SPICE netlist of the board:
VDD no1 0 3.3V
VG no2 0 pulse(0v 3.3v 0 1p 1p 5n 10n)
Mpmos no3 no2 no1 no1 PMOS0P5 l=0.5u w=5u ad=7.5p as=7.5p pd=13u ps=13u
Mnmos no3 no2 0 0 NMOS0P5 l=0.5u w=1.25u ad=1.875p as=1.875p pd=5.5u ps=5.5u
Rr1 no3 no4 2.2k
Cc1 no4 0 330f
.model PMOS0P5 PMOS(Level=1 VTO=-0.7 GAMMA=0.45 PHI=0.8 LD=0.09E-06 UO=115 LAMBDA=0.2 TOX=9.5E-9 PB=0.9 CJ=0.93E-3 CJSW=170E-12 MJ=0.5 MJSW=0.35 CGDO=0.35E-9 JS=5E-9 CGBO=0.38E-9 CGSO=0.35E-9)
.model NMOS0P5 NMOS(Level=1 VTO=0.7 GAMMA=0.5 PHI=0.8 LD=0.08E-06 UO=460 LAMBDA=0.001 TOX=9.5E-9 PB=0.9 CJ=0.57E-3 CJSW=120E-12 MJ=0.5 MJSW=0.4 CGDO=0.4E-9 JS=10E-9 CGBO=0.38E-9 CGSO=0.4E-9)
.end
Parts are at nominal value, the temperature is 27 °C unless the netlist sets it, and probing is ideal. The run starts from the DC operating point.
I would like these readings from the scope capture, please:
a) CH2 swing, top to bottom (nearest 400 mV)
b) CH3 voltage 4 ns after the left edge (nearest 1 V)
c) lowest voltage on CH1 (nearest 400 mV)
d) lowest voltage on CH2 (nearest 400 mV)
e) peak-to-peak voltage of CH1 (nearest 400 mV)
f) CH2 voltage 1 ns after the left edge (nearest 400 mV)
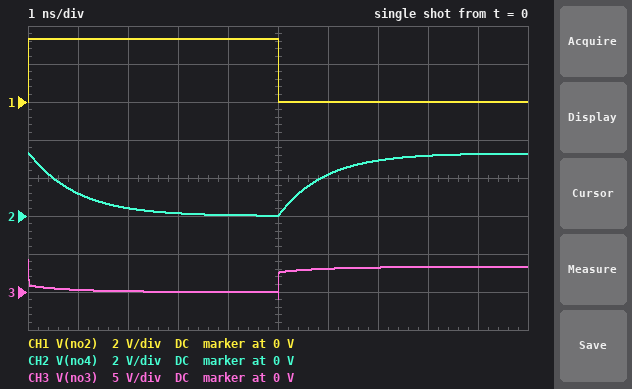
3.2 V
0 V
0 V
0 V
3.2 V
1.2 V
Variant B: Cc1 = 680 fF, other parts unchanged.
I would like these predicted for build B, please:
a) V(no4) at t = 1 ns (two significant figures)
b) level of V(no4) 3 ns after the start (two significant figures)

2.0 V
720 mV
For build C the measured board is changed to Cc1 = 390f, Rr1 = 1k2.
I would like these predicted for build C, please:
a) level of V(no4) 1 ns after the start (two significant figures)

900 mV
